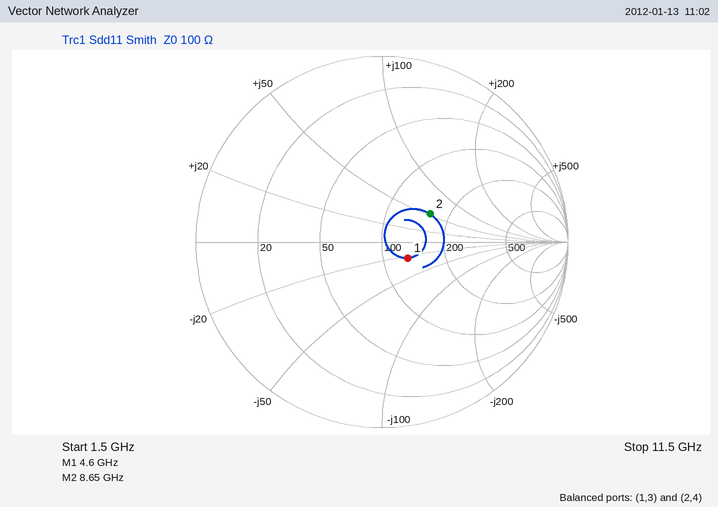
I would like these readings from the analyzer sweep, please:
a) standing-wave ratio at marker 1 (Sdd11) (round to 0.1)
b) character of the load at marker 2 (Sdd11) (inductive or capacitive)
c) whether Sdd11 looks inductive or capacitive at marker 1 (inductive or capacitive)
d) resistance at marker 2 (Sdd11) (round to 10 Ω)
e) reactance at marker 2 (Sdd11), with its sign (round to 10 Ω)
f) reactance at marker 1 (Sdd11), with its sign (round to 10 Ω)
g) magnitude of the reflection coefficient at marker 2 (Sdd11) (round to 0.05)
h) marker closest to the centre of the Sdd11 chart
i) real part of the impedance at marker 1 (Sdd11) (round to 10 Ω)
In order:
1.4
inductive
capacitive
160 Ω
+50 Ω
-20 Ω
0.30
marker 1
130 Ω
